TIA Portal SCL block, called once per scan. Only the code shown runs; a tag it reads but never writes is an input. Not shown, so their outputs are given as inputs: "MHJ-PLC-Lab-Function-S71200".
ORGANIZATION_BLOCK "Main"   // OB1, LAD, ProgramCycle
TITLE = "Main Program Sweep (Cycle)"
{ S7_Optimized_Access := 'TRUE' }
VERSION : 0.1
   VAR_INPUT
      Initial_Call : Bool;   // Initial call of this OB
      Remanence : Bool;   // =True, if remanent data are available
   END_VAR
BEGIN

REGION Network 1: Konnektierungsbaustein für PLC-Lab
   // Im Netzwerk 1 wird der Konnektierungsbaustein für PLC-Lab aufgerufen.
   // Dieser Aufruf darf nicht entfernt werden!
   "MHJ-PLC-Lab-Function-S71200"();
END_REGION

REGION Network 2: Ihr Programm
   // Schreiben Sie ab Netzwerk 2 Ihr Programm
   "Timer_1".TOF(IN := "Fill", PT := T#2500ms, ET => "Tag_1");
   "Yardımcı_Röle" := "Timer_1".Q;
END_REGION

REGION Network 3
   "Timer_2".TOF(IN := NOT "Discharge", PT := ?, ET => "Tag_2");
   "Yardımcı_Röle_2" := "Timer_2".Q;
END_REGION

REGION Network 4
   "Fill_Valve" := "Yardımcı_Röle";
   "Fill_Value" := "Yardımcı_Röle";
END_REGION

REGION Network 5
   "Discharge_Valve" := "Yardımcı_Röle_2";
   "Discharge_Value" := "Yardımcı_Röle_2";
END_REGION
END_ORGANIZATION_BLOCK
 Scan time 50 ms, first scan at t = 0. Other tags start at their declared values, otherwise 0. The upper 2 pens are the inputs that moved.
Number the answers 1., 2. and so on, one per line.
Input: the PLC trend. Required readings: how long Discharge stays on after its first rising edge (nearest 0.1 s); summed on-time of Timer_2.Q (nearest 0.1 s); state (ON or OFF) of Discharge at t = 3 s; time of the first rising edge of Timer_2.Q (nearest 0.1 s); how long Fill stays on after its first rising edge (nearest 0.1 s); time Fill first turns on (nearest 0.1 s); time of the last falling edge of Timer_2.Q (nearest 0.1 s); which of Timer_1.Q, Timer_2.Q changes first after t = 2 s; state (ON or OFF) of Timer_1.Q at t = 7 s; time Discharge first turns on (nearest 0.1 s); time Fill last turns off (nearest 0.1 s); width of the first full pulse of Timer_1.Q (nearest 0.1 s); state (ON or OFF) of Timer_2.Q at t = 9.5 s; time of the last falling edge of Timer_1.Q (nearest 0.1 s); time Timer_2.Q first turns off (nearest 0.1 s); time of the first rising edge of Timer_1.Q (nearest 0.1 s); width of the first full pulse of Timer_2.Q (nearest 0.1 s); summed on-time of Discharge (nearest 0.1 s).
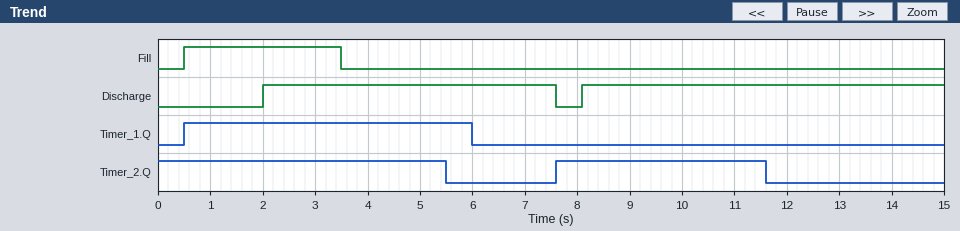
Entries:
1. 5.6 s
2. 9.5 s
3. ON
4. 7.6 s
5. 3.0 s
6. 0.5 s
7. 11.6 s
8. Timer_2.Q
9. OFF
10. 2.0 s
11. 3.5 s
12. 5.5 s
13. ON
14. 6.0 s
15. 5.5 s
16. 0.5 s
17. 4.0 s
18. 12.5 s
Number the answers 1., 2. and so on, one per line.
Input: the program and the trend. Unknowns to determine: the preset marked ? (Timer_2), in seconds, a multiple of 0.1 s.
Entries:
1. 3.5 s
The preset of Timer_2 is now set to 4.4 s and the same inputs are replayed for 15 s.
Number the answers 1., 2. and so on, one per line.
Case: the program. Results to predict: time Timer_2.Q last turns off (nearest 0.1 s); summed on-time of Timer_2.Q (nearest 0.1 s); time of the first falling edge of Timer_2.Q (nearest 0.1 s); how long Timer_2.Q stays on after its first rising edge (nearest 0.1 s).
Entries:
1. 12.5 s
2. 11.3 s
3. 6.4 s
4. 4.9 s
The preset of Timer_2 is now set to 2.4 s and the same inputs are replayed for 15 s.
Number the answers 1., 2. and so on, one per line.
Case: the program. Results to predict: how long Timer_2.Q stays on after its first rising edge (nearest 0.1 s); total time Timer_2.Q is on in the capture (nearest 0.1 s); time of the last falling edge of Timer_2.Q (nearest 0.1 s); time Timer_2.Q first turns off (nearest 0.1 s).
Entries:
1. 2.9 s
2. 7.3 s
3. 10.5 s
4. 4.4 s
